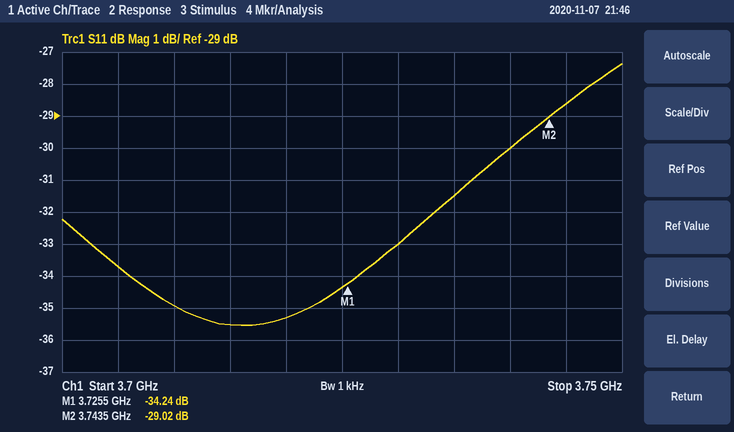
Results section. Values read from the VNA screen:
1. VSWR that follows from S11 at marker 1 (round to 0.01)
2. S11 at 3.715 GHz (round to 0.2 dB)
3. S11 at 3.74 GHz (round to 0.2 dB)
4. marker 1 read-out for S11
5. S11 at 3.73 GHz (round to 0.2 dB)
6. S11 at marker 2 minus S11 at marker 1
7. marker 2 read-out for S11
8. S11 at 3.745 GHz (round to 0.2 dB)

1.04
-35.6 dB
-30.0 dB
-34.24 dB
-33.0 dB
5.22 dB
-29.02 dB
-28.6 dB
